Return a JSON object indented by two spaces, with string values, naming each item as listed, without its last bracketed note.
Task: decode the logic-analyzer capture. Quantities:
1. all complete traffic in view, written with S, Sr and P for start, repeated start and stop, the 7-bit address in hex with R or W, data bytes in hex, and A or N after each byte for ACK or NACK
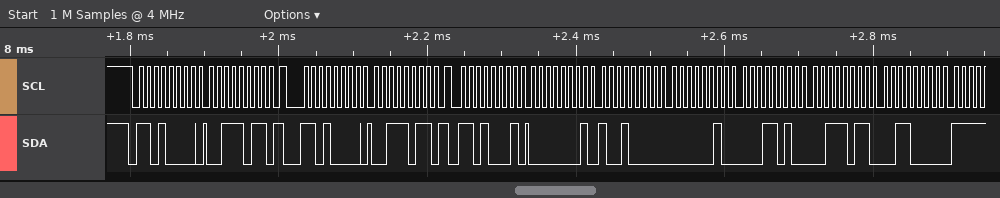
{
  "all complete traffic in view, written with S, Sr and P for start, repeated start and stop, the 7-bit address in hex with R or W, data bytes in hex, and A or N after each byte for ACK or NACK": "S 68W A 3B A Sr 68W A 3B A Sr 68R A 01 A 90 A 02 A 1A A 3B A 30 A"
}
